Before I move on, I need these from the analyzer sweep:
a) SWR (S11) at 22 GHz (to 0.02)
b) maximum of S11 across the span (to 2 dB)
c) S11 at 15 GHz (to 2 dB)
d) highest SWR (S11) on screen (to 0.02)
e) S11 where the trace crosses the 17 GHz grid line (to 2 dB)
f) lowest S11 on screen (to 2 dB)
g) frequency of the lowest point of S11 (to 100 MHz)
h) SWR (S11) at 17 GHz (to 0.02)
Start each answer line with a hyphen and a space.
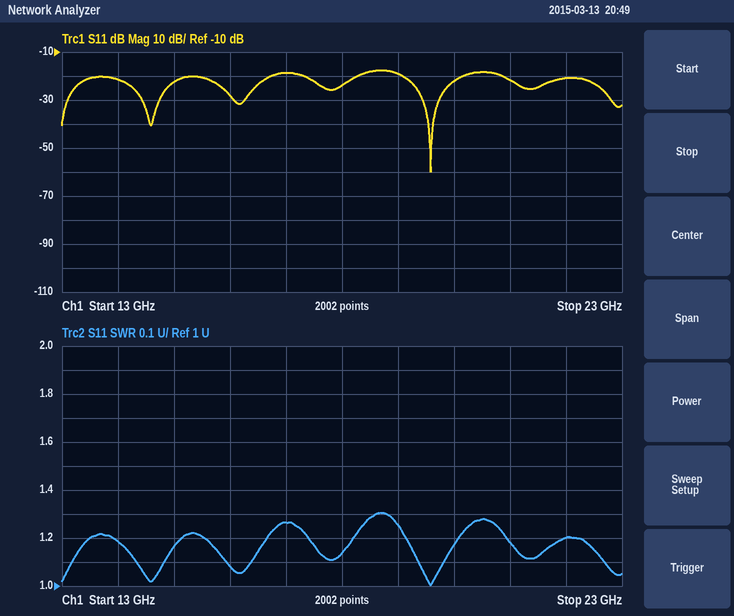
- 1.20
- -18 dB
- -22 dB
- 1.30
- -18 dB
- -60 dB
- 19.6 GHz
- 1.26
